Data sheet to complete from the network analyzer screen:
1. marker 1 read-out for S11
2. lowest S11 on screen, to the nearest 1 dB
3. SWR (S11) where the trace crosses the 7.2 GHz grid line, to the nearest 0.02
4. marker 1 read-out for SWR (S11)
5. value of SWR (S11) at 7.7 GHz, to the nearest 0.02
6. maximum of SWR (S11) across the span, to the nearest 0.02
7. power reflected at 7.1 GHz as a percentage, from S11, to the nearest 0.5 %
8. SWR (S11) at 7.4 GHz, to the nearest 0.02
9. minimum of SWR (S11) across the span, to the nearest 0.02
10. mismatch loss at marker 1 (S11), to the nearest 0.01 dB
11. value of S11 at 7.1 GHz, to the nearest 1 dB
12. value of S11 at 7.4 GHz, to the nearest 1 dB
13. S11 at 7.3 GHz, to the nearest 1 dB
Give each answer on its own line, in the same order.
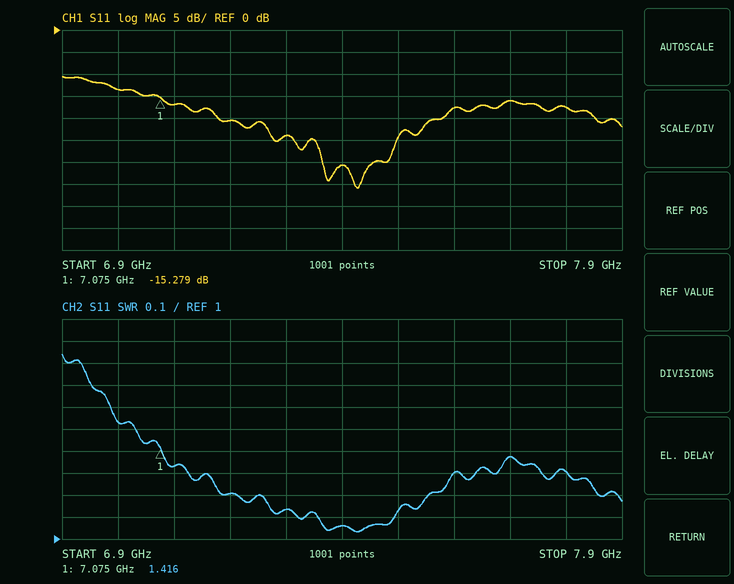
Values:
-15.279 dB
-36 dB
1.20
1.416
1.38
1.84
2.0 %
1.06
1.04
0.13 dB
-17 dB
-31 dB
-24 dB
